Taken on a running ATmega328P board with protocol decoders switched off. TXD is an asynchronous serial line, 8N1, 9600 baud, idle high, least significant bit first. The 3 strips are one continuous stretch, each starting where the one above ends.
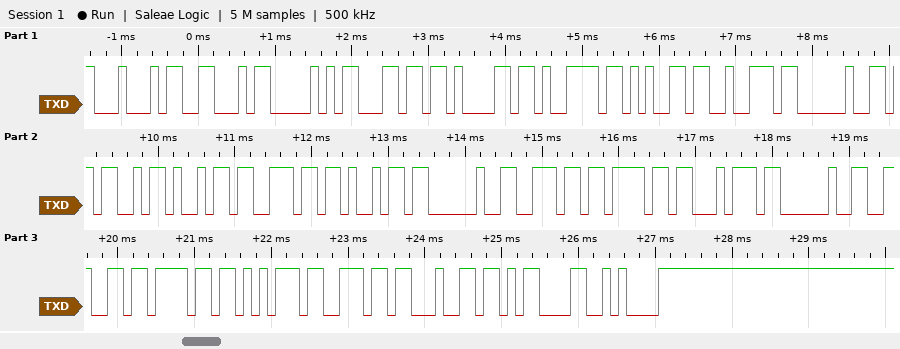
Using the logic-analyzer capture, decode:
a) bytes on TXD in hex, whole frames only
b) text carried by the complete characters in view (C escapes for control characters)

44 46 50 6C 61 79 65 72 20 4D 69 6E 69 20 6E 6F 74 20 66 6F 75 6E 64 0D 0A
"DFPlayer Mini not found\r\n"
